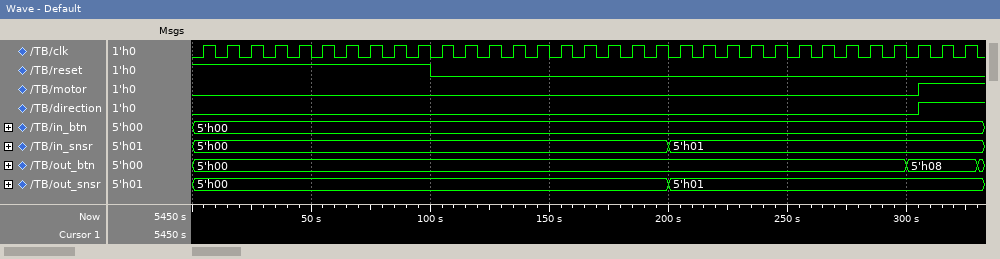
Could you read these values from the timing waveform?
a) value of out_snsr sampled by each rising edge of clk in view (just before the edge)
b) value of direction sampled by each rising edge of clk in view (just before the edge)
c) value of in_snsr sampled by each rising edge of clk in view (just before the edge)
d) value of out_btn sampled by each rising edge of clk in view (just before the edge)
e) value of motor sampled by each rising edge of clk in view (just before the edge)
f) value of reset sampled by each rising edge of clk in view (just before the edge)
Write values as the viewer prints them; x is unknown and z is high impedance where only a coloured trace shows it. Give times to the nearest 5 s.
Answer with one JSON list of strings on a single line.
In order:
["5'h00, 5'h00, 5'h00, 5'h00, 5'h00, 5'h00, 5'h00, 5'h00, 5'h00, 5'h00, 5'h00, 5'h00, 5'h00, 5'h00, 5'h00, 5'h00, 5'h00, 5'h00, 5'h00, 5'h00, 5'h01, 5'h01, 5'h01, 5'h01, 5'h01, 5'h01, 5'h01, 5'h01, 5'h01, 5'h01, 5'h01, 5'h01, 5'h01", "0 0 0 0 0 0 0 0 0 0 0 0 0 0 0 0 0 0 0 0 0 0 0 0 0 0 0 0 0 0 0 1 1", "5'h00, 5'h00, 5'h00, 5'h00, 5'h00, 5'h00, 5'h00, 5'h00, 5'h00, 5'h00, 5'h00, 5'h00, 5'h00, 5'h00, 5'h00, 5'h00, 5'h00, 5'h00, 5'h00, 5'h00, 5'h01, 5'h01, 5'h01, 5'h01, 5'h01, 5'h01, 5'h01, 5'h01, 5'h01, 5'h01, 5'h01, 5'h01, 5'h01", "5'h00, 5'h00, 5'h00, 5'h00, 5'h00, 5'h00, 5'h00, 5'h00, 5'h00, 5'h00, 5'h00, 5'h00, 5'h00, 5'h00, 5'h00, 5'h00, 5'h00, 5'h00, 5'h00, 5'h00, 5'h00, 5'h00, 5'h00, 5'h00, 5'h00, 5'h00, 5'h00, 5'h00, 5'h00, 5'h00, 5'h08, 5'h08, 5'h08", "0 0 0 0 0 0 0 0 0 0 0 0 0 0 0 0 0 0 0 0 0 0 0 0 0 0 0 0 0 0 0 1 1", "1 1 1 1 1 1 1 1 1 1 0 0 0 0 0 0 0 0 0 0 0 0 0 0 0 0 0 0 0 0 0 0 0"]
